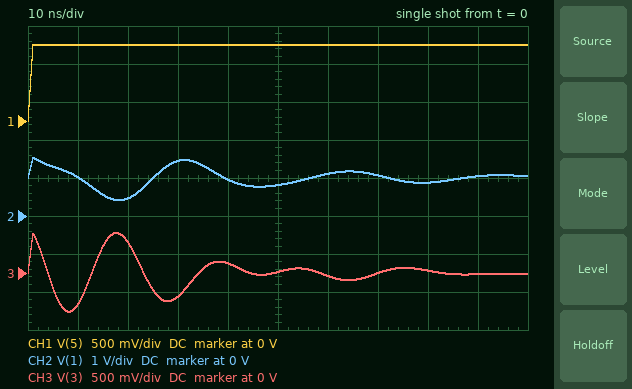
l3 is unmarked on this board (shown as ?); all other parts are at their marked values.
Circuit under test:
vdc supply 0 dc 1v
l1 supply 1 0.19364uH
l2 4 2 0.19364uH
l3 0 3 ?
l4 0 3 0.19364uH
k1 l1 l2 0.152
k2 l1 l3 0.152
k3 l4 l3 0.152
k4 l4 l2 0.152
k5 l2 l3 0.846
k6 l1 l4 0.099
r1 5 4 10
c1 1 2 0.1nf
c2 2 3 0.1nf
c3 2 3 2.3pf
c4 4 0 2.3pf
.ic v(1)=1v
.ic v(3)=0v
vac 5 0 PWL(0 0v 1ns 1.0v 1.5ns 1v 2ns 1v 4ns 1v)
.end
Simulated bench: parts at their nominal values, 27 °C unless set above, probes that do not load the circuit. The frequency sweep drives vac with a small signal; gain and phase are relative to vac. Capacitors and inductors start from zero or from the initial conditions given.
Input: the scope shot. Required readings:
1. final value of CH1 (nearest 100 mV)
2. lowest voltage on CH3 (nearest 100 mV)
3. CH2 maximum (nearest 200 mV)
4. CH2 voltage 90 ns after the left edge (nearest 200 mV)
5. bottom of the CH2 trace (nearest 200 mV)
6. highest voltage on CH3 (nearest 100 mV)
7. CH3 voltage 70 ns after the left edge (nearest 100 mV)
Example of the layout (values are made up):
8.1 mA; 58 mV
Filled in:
1.0 V; -500 mV; 1.6 V; 1.0 V; 400 mV; 500 mV; 0 V
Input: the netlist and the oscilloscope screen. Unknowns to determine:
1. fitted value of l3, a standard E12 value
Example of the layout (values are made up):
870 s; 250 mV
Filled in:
470 nH
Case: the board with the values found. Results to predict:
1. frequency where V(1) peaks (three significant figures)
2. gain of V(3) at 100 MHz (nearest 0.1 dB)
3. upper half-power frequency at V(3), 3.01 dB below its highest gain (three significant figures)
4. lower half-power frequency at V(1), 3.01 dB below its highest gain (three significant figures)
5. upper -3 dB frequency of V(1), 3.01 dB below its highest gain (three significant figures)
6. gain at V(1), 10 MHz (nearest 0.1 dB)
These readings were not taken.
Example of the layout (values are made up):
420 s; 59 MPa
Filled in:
32.6 MHz; -1.3 dB; 61.9 MHz; 29.1 MHz; 38.3 MHz; -22.0 dB
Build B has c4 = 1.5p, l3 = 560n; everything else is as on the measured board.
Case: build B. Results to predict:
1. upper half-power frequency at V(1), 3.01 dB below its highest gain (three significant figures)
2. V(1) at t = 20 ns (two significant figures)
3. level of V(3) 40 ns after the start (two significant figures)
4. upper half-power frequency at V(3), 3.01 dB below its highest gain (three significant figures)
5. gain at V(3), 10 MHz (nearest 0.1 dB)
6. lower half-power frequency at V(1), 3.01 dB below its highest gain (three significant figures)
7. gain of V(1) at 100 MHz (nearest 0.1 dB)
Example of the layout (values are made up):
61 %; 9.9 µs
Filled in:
38.8 MHz; 480 mV; 220 mV; 58.5 MHz; -42.9 dB; 29.4 MHz; -4.2 dB
